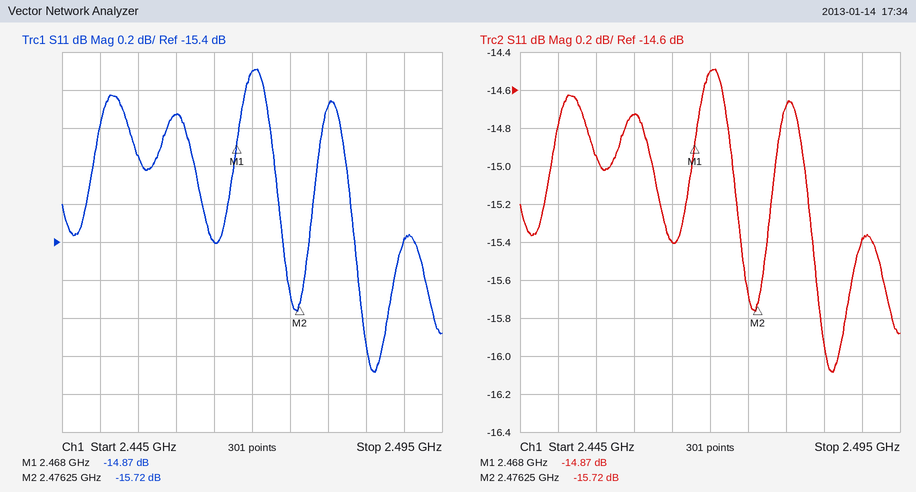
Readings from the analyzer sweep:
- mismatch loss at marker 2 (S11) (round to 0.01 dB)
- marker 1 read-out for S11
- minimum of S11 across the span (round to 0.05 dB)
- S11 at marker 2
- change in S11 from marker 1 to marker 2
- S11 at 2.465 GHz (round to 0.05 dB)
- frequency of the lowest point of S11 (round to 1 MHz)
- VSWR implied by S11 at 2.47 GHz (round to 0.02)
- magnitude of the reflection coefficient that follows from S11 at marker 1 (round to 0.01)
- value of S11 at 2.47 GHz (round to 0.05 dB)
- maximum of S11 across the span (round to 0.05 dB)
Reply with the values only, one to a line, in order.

0.12 dB
-14.87 dB
-16.10 dB
-15.72 dB
-0.85 dB
-15.40 dB
2.486 GHz
1.46
0.18
-14.50 dB
-14.50 dB
